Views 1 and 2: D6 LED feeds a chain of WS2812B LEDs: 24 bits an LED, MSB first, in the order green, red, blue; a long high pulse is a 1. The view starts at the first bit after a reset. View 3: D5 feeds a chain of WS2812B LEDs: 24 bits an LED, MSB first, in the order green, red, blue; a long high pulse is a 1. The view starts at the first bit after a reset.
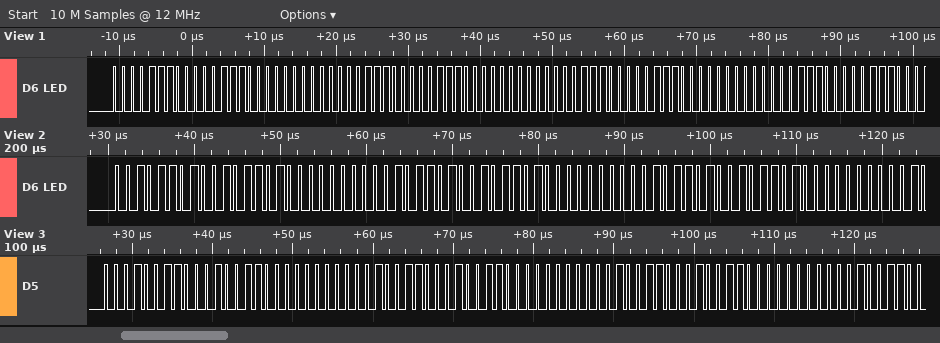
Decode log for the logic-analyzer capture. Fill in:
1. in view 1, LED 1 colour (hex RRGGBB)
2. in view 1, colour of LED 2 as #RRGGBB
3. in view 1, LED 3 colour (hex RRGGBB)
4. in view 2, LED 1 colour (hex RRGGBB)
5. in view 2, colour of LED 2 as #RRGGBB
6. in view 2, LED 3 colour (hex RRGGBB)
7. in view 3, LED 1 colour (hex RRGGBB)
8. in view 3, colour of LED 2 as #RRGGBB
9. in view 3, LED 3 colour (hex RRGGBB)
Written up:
#0E0E00
#0E0E00
#0E0E00
#2D2D00
#2D2D00
#2D2D00
#131300
#131300
#131300
